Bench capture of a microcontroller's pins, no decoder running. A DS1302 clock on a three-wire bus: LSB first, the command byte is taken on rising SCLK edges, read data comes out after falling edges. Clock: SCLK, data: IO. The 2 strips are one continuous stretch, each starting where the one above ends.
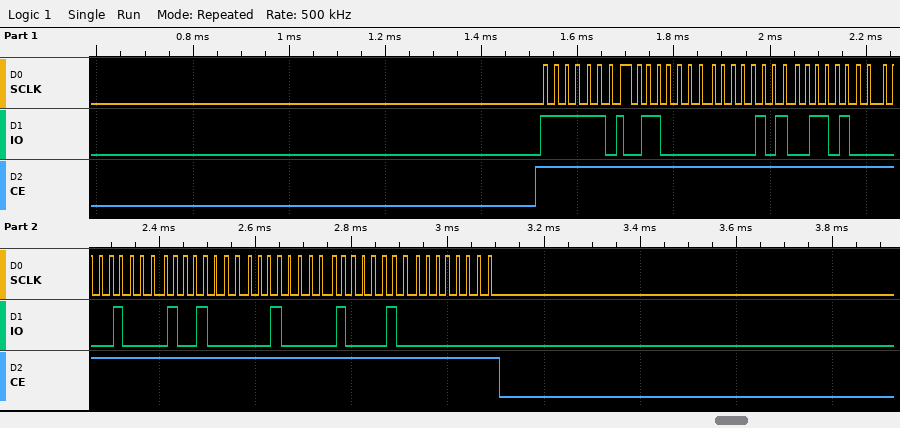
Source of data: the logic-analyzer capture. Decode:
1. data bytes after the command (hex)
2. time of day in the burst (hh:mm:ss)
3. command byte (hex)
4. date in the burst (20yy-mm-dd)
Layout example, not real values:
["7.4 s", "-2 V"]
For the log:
["06 50 16 08 09 04 21 00", "16:50:06", "0xBF", "2021-09-08"]
